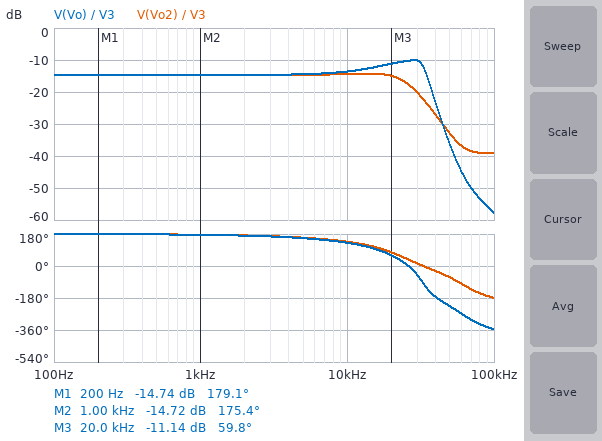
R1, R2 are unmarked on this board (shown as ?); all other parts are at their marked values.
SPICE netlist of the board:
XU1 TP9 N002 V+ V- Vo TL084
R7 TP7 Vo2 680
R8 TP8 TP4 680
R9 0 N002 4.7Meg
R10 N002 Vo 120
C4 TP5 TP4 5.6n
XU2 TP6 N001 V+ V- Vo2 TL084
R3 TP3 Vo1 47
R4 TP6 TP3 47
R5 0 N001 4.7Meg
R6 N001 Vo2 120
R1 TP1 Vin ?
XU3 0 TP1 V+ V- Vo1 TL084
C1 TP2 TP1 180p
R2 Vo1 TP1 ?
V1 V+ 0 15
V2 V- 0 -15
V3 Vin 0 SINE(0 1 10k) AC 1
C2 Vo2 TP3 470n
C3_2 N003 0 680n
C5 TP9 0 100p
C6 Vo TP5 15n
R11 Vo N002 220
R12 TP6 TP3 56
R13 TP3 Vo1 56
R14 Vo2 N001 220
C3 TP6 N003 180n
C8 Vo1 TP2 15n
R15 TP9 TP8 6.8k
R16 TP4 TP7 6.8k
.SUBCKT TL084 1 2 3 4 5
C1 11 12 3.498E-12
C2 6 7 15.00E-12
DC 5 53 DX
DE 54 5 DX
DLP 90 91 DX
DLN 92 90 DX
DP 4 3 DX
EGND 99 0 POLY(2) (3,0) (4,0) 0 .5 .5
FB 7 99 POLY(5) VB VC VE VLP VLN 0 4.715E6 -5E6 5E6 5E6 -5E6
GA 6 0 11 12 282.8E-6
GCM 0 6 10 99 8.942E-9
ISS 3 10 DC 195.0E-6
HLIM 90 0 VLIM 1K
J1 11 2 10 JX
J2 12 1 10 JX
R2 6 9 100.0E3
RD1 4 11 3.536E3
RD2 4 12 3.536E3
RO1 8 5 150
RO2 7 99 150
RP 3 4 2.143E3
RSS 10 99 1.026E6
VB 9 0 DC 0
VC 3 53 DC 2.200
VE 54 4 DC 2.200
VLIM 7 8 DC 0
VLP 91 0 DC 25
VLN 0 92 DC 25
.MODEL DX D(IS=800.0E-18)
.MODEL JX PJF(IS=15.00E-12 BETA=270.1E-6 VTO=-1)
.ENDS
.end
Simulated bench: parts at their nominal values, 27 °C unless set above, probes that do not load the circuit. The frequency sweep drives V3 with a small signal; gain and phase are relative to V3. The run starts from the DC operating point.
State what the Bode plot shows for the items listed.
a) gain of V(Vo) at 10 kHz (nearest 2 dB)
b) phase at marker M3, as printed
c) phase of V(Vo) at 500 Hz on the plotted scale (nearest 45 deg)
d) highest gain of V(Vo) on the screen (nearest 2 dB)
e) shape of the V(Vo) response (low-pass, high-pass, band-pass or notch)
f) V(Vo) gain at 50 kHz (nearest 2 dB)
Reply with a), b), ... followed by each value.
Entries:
a) -14 dB
b) 59.8 deg
c) 180 deg
d) -10 dB
e) low-pass
f) -36 dB
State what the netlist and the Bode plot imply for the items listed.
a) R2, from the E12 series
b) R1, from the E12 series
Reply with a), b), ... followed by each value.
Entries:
a) 22 kΩ
b) 120 kΩ
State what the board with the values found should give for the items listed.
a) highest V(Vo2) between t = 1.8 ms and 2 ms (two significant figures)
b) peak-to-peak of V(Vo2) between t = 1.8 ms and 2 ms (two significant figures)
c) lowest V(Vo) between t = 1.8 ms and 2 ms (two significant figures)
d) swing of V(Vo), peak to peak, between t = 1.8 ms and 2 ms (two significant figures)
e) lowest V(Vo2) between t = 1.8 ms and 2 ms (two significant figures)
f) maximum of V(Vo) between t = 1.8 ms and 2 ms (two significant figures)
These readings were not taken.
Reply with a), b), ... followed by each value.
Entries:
a) 190 mV
b) 380 mV
c) -210 mV
d) 420 mV
e) -190 mV
f) 210 mV
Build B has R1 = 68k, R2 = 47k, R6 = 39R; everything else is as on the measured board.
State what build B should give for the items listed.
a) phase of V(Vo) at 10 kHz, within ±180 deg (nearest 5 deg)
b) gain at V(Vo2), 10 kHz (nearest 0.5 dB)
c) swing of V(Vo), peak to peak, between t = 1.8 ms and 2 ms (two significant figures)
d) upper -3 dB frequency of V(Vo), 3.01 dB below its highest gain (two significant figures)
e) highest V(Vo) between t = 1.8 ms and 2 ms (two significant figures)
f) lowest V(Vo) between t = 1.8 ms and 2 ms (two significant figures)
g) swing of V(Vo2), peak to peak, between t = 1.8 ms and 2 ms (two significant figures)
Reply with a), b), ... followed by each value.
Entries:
a) 115 deg
b) -3.5 dB
c) 1.4 V
d) 33 kHz
e) 720 mV
f) -720 mV
g) 1.3 V
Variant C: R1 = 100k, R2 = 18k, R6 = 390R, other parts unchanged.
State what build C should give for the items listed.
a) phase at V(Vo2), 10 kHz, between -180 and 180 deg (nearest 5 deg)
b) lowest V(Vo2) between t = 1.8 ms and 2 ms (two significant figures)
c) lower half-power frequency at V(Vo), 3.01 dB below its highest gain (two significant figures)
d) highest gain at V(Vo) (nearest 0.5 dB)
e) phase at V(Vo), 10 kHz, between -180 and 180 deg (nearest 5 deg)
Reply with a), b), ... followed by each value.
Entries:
a) 140 deg
b) -190 mV
c) 14 kHz
d) -9.5 dB
e) 135 deg
